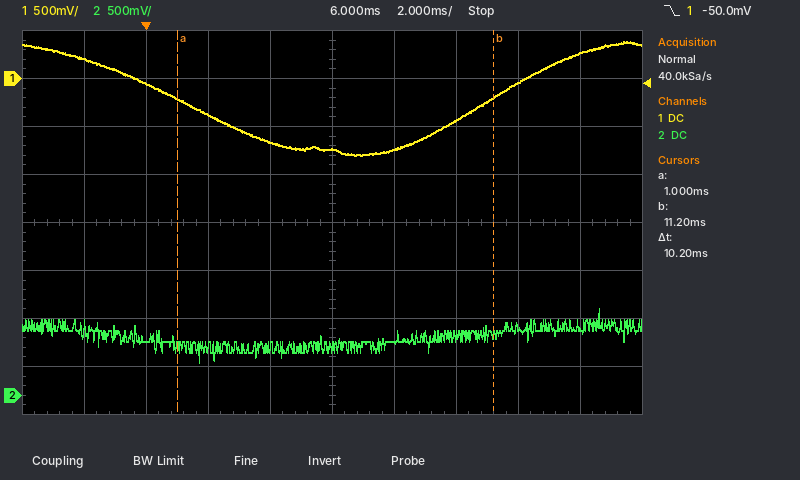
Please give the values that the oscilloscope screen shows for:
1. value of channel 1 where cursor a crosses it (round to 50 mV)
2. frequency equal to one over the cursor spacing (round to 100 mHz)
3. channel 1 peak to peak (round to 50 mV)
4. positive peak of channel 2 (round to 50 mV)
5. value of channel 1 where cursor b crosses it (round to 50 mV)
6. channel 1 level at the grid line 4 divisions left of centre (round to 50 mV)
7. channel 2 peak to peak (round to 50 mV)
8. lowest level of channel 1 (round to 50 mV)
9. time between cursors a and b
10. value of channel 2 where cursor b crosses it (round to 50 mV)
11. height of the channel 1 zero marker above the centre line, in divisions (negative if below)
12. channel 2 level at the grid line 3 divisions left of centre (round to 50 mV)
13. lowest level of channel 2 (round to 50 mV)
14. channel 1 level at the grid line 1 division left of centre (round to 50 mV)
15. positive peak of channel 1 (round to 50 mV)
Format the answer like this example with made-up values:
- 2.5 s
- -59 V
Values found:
- -200 mV
- 98.0 Hz
- 1.20 V
- 900 mV
- -200 mV
- 200 mV
- 550 mV
- -800 mV
- 10.2 ms
- 650 mV
- +3.0 div
- 550 mV
- 350 mV
- -650 mV
- 400 mV
